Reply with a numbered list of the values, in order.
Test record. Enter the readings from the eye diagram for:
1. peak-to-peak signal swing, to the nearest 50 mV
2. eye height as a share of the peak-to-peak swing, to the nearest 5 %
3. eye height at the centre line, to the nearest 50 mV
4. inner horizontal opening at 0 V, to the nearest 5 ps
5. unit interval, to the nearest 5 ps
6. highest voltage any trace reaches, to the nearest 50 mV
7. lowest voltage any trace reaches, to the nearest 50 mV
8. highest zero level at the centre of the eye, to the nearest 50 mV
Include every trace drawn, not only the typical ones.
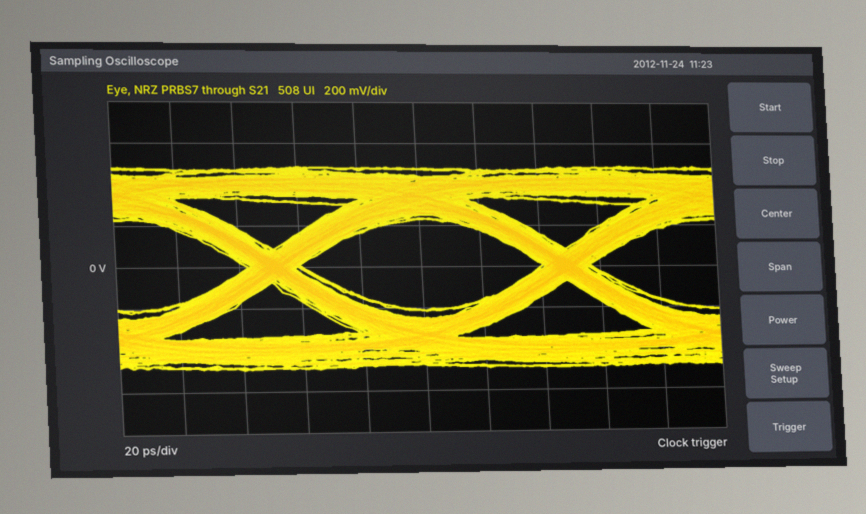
1. 1.00 V
2. 45 %
3. 450 mV
4. 80 ps
5. 95 ps
6. 500 mV
7. -500 mV
8. -200 mV
